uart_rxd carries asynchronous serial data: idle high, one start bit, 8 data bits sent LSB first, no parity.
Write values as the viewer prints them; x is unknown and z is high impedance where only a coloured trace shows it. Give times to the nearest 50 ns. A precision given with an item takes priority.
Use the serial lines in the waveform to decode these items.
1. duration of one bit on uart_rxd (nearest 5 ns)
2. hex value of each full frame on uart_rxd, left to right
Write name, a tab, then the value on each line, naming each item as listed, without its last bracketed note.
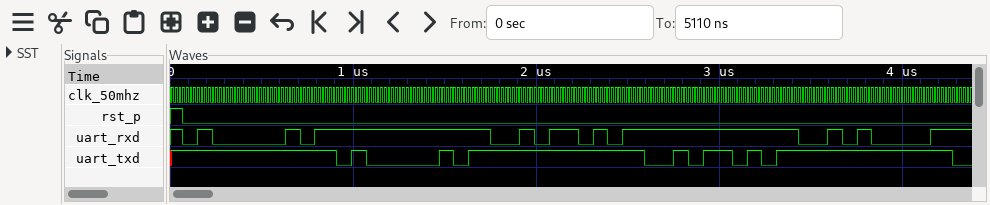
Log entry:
duration of one bit on uart_rxd	80 ns
hex value of each full frame on uart_rxd, left to right	41, 5A, 0A
